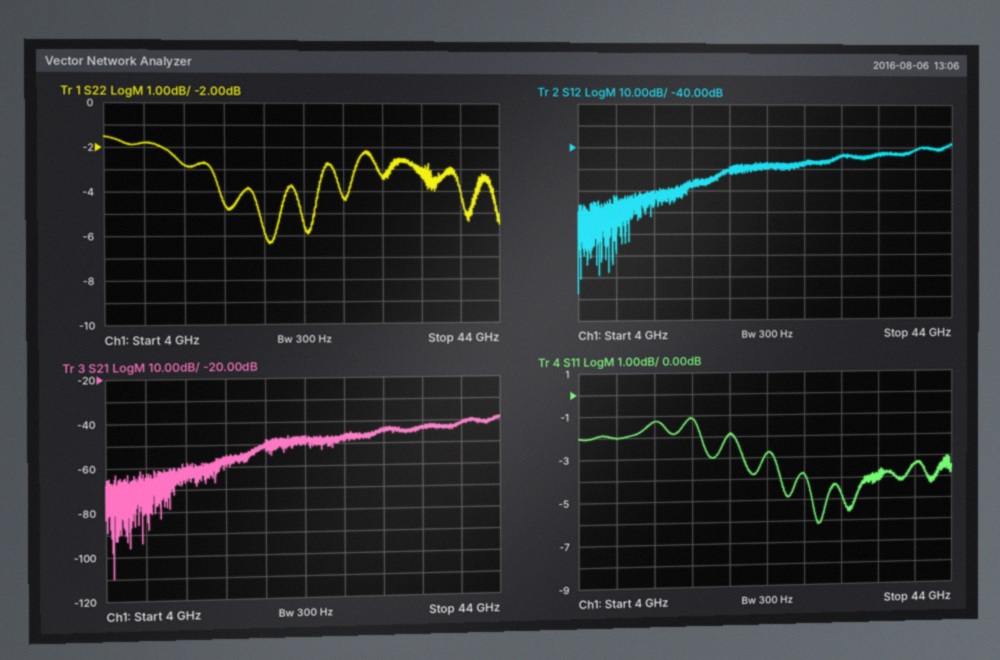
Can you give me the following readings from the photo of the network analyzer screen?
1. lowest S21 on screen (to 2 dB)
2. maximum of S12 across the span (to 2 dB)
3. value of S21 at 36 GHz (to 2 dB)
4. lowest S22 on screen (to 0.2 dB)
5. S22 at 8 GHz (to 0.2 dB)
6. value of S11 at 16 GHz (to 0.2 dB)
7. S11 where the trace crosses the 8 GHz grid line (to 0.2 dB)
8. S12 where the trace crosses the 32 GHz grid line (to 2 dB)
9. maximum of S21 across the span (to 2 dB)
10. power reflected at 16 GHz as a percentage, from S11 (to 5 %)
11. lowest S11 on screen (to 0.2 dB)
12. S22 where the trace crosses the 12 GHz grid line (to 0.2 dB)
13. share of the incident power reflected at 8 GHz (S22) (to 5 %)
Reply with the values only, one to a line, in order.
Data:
-110 dB
-38 dB
-44 dB
-6.4 dB
-1.8 dB
-1.2 dB
-2.0 dB
-44 dB
-38 dB
75 %
-6.2 dB
-2.8 dB
65 %
